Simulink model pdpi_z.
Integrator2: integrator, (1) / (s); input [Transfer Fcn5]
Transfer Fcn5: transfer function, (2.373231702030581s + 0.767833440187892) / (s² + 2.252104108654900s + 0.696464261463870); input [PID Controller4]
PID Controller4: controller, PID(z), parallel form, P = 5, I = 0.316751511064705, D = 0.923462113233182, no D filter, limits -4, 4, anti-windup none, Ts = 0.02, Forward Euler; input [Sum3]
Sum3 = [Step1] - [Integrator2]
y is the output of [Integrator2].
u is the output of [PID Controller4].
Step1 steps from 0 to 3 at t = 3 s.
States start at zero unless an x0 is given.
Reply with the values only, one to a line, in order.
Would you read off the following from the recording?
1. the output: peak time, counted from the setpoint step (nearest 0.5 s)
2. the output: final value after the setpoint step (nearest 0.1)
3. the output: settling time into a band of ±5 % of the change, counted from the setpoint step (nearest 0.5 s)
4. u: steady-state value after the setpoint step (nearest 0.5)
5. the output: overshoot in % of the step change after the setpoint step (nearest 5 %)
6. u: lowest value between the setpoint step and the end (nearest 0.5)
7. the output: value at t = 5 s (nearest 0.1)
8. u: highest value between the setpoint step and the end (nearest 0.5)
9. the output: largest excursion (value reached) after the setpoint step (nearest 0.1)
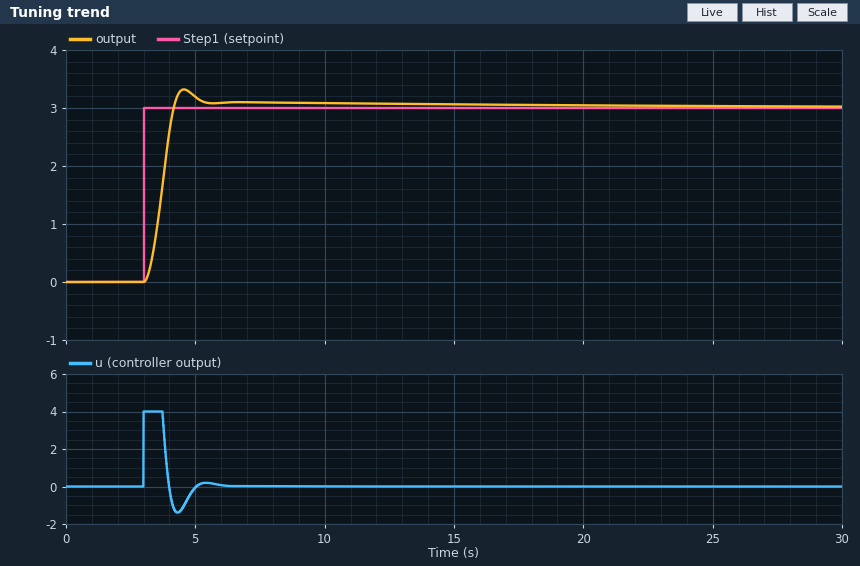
1.5 s
3.0
2.0 s
0.0
10 %
-1.5
3.2
4.0
3.3
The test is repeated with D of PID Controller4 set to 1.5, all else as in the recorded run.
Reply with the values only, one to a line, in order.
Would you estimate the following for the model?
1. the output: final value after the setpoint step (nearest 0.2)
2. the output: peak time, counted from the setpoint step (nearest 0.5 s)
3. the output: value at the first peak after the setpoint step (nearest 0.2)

3.0
2.0 s
3.2
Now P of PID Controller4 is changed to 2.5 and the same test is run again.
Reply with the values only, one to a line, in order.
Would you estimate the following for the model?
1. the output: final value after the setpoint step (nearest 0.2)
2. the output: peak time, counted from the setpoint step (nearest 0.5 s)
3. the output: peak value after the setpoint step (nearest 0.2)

3.0
2.5 s
3.2
